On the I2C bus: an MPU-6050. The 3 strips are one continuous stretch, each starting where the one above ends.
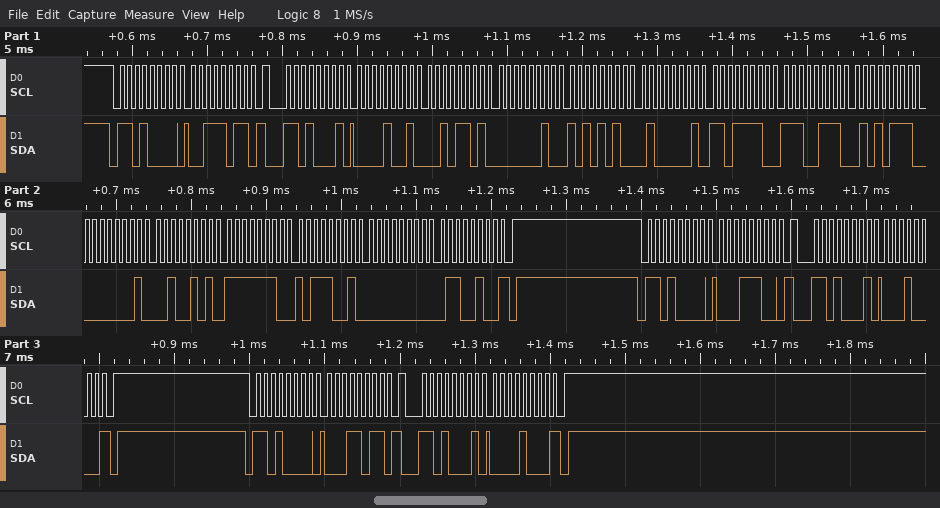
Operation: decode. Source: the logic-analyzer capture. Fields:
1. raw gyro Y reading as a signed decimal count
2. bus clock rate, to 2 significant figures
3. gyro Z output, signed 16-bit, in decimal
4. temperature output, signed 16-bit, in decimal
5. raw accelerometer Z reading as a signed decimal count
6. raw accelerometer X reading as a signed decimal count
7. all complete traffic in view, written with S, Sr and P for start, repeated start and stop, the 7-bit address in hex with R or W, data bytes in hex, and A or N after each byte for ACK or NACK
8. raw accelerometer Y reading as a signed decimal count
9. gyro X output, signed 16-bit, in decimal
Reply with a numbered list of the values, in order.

1. -327
2. 100 kHz
3. 100
4. -6313
5. 16862
6. 2349
7. S 68W A 3B A Sr 68R A 09 A 2D A 02 A AA A 41 A DE A E7 A 57 A 01 A 25 A FE A B9 A 00 A 64 N P S 68W A 1C A Sr 68R A 10 N P S 68W A 1B A Sr 68R A 08 N P
8. 682
9. 293
